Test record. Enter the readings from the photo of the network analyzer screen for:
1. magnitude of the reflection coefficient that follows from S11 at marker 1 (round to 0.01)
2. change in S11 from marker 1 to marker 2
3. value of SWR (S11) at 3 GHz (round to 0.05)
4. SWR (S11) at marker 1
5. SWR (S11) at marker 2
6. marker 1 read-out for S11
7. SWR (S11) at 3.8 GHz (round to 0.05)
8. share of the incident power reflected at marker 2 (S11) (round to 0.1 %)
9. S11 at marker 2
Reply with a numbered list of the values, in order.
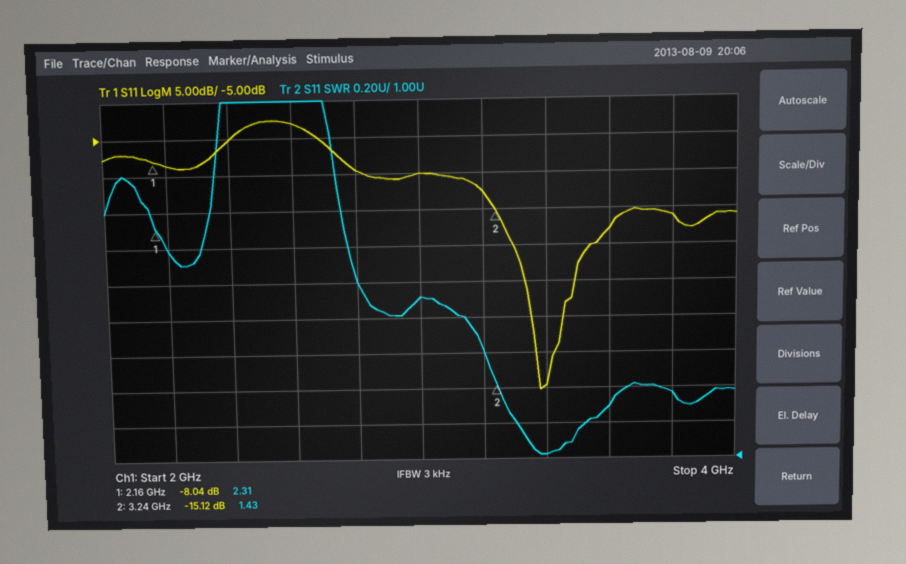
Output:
1. 0.40
2. -7.08 dB
3. 1.90
4. 2.31
5. 1.43
6. -8.04 dB
7. 1.35
8. 3.1 %
9. -15.12 dB
